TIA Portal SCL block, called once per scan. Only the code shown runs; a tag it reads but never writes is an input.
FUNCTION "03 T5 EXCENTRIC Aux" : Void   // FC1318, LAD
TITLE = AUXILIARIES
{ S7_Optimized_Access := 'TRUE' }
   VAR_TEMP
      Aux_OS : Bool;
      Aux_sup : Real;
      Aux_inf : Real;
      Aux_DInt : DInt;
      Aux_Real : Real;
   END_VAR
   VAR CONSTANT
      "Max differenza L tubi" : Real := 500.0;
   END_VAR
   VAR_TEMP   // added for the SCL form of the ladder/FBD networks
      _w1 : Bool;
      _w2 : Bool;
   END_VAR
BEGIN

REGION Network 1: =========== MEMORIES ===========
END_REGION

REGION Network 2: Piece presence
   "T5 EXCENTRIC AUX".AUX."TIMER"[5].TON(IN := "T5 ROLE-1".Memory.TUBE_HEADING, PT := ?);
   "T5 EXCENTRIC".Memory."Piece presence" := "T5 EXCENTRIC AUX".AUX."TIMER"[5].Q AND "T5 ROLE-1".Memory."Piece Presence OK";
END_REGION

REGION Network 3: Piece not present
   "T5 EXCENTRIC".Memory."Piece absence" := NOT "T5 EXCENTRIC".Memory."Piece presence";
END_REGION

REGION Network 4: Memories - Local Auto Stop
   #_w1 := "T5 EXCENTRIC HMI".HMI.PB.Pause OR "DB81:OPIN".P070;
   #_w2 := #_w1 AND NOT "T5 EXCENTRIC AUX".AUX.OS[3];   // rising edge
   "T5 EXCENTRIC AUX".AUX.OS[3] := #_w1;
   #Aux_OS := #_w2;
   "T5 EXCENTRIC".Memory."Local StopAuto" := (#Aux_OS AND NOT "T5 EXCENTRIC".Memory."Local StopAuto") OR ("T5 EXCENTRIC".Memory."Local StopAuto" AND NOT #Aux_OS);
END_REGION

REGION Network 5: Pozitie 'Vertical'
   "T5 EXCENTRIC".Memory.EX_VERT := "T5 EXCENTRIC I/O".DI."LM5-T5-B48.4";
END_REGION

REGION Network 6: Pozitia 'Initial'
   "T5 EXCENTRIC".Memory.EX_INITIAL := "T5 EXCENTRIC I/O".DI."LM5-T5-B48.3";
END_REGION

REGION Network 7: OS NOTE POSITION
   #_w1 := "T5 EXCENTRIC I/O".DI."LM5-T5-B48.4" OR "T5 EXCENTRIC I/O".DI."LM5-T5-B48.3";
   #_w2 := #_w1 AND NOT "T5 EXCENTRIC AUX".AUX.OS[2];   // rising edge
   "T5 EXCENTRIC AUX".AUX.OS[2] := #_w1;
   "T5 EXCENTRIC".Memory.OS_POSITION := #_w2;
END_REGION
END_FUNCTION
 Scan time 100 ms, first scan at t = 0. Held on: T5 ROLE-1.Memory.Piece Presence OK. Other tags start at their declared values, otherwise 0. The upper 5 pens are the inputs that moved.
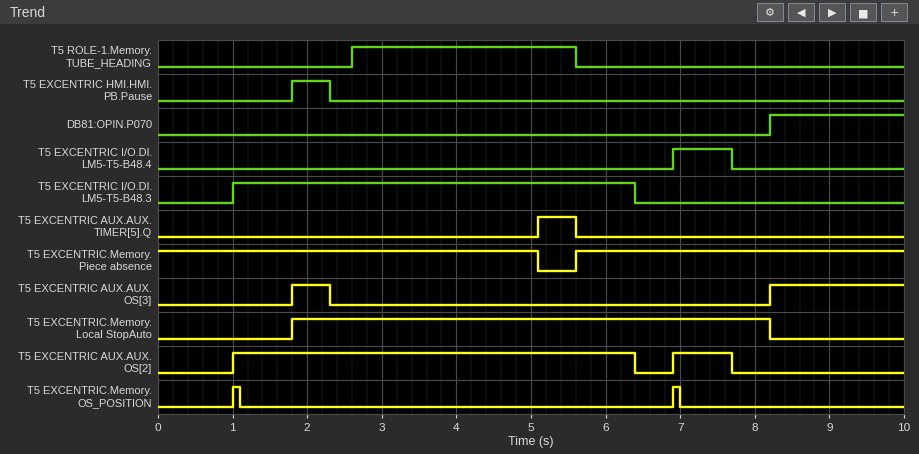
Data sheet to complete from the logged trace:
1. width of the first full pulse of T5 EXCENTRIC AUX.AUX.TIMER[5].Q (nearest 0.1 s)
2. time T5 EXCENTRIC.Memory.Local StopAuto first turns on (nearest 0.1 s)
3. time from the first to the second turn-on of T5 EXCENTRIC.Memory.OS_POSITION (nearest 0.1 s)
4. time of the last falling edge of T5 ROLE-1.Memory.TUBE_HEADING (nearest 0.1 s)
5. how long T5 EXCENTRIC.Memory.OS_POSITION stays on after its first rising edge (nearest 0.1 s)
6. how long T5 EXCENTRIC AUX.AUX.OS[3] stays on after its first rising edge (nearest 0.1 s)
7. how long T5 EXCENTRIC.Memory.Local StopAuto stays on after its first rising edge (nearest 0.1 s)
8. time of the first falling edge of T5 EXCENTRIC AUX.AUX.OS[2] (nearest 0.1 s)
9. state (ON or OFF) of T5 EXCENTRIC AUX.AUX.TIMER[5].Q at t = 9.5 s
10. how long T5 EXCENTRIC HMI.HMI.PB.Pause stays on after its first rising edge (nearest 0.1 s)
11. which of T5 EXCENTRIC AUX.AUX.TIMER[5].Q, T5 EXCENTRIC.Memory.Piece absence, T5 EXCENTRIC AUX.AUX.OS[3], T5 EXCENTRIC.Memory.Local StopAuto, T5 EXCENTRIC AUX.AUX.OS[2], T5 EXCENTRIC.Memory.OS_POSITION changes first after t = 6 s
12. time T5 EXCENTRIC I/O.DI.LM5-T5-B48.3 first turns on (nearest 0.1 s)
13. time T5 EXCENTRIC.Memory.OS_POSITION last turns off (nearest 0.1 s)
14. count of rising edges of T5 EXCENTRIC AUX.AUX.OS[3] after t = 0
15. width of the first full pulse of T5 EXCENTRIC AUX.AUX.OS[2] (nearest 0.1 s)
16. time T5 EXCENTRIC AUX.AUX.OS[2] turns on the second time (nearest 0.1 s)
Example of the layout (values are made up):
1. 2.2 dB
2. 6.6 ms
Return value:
1. 0.5 s
2. 1.8 s
3. 5.9 s
4. 5.6 s
5. 0.1 s
6. 0.5 s
7. 6.4 s
8. 6.4 s
9. OFF
10. 0.5 s
11. T5 EXCENTRIC AUX.AUX.OS[2]
12. 1.0 s
13. 7.0 s
14. 2
15. 5.4 s
16. 6.9 s
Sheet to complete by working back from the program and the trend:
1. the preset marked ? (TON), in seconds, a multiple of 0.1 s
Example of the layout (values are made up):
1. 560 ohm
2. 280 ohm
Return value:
1. 2.5 s
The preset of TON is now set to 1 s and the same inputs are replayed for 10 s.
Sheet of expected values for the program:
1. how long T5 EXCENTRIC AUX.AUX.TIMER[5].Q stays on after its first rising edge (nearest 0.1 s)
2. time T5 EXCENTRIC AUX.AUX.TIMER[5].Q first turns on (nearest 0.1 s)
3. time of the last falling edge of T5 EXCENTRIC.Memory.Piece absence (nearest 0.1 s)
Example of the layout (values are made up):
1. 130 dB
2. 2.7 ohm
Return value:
1. 2.0 s
2. 3.6 s
3. 3.6 s
